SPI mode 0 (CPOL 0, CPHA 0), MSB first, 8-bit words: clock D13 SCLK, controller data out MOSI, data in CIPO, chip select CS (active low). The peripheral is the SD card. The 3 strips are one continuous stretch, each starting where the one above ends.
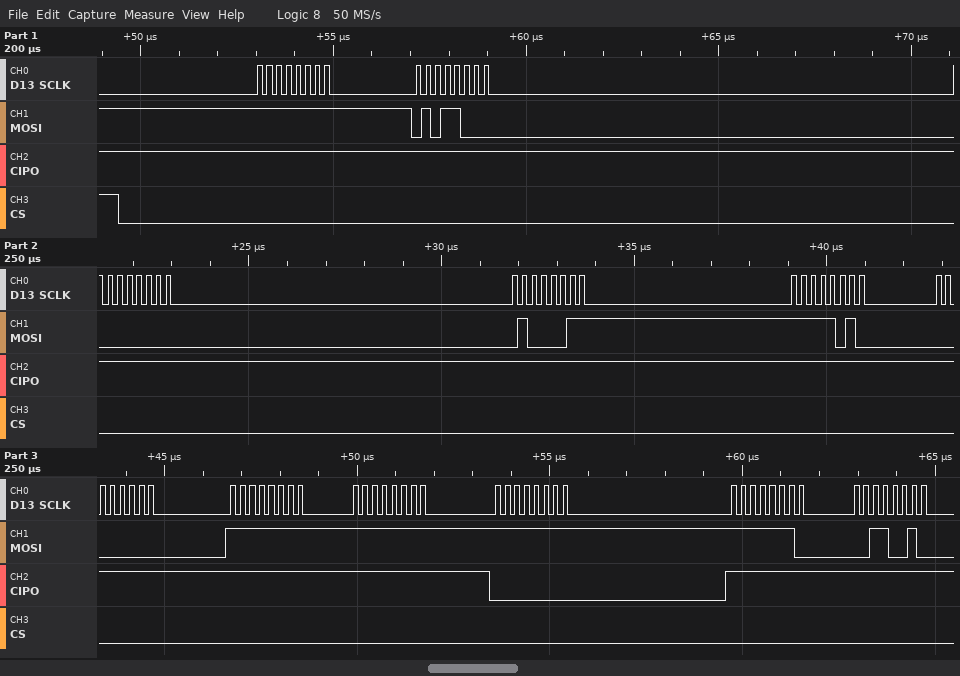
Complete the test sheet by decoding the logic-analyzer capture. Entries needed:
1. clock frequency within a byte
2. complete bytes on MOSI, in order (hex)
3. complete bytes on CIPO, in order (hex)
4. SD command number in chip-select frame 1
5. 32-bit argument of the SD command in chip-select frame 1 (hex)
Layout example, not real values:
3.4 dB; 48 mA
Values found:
4 MHz; 0xFF 0x58 0x00 0x43 0xFA 0x00 0xFF 0xFF 0xFF 0xFE 0x32; 0xFF 0xFF 0xFF 0xFF 0xFF 0xFF 0xFF 0xFF 0x00 0xFF 0xFF; CMD24; 0x0043FA00
